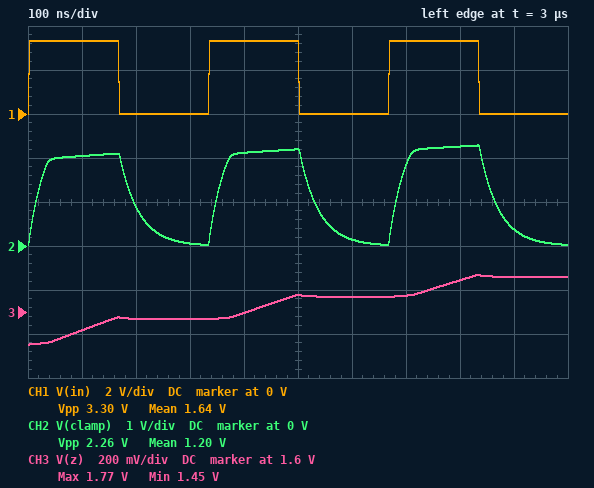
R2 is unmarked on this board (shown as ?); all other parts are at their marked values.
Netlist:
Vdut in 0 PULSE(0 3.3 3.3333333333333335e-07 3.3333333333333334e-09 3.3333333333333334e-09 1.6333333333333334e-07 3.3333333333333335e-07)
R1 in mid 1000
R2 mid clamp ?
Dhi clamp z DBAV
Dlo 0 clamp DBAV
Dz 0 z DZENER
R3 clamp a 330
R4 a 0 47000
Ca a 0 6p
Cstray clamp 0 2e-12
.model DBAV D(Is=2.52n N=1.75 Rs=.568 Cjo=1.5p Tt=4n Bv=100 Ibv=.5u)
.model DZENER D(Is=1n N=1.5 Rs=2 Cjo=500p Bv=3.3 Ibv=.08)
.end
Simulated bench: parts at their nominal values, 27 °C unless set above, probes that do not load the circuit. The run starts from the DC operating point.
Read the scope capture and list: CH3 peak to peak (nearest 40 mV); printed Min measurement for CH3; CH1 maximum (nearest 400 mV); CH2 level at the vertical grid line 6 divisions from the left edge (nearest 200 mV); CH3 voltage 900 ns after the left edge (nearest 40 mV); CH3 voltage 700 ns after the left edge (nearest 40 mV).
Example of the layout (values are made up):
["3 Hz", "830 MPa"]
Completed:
["320 mV", "1.45 V", "3.2 V", "200 mV", "1.76 V", "1.68 V"]
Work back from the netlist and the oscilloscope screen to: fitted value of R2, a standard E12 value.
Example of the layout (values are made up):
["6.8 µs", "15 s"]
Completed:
["2.7 kΩ"]
